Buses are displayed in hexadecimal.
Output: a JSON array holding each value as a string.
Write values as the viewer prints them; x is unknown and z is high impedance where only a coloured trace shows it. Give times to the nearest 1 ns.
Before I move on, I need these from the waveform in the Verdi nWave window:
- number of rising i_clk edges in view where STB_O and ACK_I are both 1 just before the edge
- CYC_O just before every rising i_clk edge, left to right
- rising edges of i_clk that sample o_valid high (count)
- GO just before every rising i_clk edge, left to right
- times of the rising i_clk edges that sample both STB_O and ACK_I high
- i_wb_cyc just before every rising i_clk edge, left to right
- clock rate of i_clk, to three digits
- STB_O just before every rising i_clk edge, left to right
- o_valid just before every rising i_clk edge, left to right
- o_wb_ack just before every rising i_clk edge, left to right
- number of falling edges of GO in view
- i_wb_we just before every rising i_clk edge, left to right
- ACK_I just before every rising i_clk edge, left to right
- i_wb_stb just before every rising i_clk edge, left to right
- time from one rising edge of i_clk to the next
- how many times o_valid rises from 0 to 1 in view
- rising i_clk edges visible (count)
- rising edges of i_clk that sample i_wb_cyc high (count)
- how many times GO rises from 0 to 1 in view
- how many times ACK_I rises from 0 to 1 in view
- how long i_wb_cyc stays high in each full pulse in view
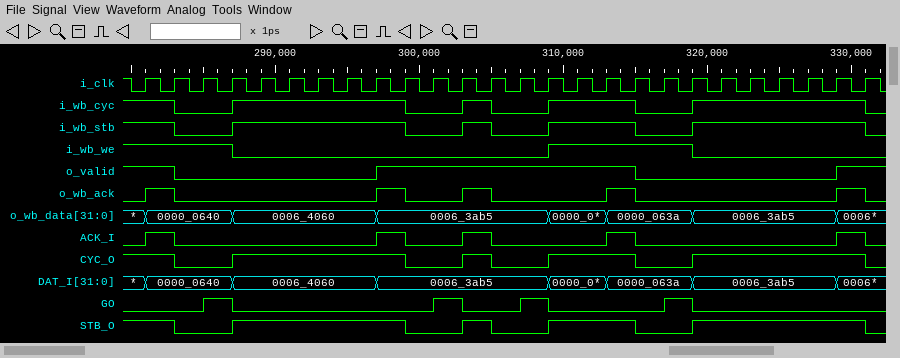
["5", "1 1 0 0 1 1 1 1 1 1 0 0 1 0 0 1 1 1 0 0 1 1 1 1 1 1", "12", "0 0 0 1 0 0 0 0 0 0 0 1 0 0 1 0 0 0 0 1 0 0 0 0 0 0", "283 ns, 299 ns, 305 ns, 315 ns, 331 ns", "1 1 0 0 1 1 1 1 1 1 0 0 1 0 0 1 1 1 0 0 1 1 1 1 1 1", "500 MHz", "1 1 0 0 1 1 1 1 1 1 0 0 1 0 0 1 1 1 0 0 1 1 1 1 1 1", "1 1 0 0 0 0 0 0 0 1 1 1 1 1 1 1 1 1 0 0 0 0 0 0 0 1", "0 1 0 0 0 0 0 0 0 1 0 0 1 0 0 0 0 1 0 0 0 0 0 0 0 1", "4", "1 1 1 1 0 0 0 0 0 0 0 0 0 0 0 1 1 1 1 1 0 0 0 0 0 0", "0 1 0 0 0 0 0 0 0 1 0 0 1 0 0 0 0 1 0 0 0 0 0 0 0 1", "1 1 0 0 1 1 1 1 1 1 0 0 1 0 0 1 1 1 0 0 1 1 1 1 1 1", "2 ns", "2", "26", "18", "4", "5", "12 ns, 2 ns, 6 ns, 12 ns"]
